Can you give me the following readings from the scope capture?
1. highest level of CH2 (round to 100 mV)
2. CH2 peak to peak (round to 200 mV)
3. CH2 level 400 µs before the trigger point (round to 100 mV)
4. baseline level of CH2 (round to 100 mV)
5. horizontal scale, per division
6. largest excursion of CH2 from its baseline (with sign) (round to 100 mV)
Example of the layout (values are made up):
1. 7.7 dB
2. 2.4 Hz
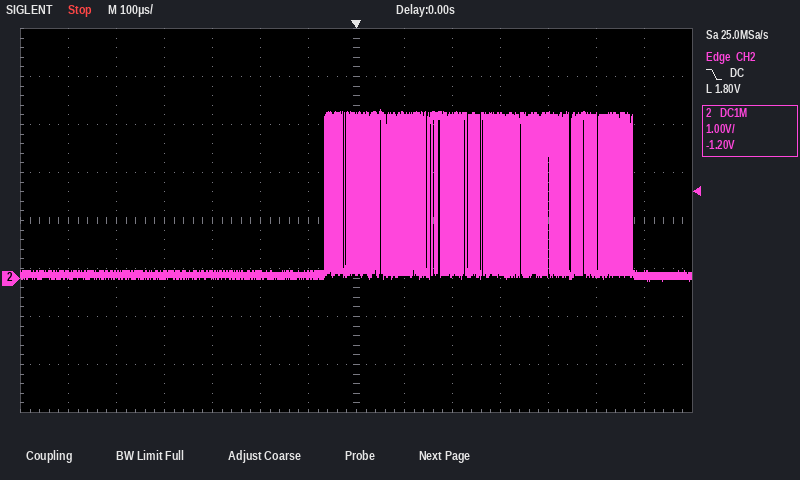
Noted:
1. 3.5 V
2. 3.6 V
3. 100 mV
4. 100 mV
5. 100 µs
6. +3.4 V
